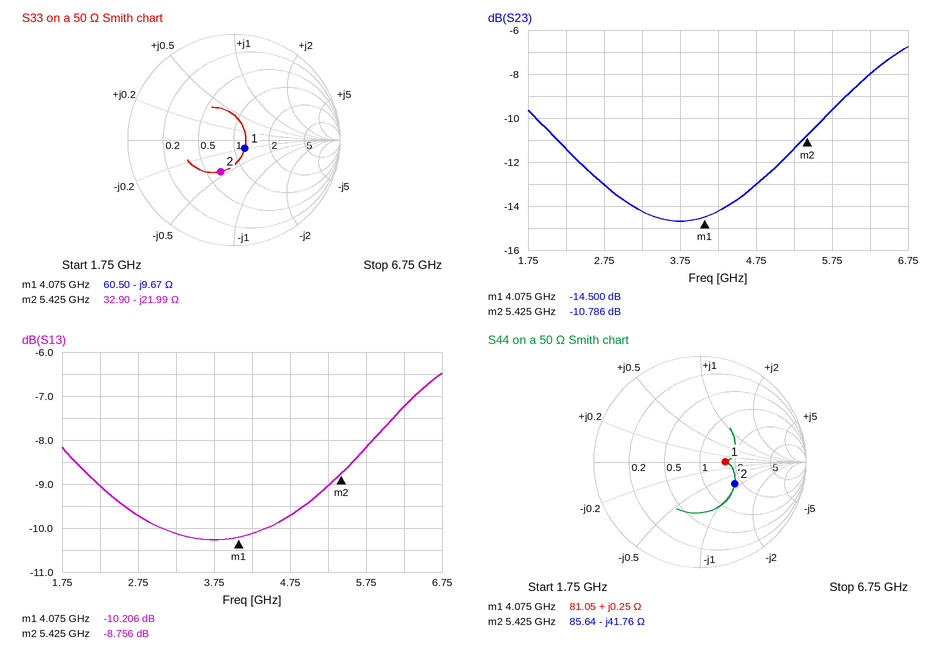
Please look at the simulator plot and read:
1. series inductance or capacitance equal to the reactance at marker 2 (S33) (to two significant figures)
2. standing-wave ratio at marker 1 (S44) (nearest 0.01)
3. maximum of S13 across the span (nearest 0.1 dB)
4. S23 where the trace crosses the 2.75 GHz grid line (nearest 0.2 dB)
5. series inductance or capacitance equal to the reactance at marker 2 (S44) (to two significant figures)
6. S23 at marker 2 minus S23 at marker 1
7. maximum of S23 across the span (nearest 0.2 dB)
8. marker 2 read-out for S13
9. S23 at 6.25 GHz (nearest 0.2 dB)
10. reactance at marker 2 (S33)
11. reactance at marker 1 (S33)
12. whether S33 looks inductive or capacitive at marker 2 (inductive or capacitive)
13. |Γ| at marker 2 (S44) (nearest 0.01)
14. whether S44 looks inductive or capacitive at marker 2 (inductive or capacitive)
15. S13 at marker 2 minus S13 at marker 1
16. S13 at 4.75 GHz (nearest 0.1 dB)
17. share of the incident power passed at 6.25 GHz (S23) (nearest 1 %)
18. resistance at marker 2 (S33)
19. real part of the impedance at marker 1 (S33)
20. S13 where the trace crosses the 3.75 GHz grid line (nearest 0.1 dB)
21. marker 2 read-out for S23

1.3 pF
1.62
-6.5 dB
-13.0 dB
700 fF
3.714 dB
-6.8 dB
-8.756 dB
-8.0 dB
-21.99 Ω
-9.67 Ω
capacitive
0.39
capacitive
1.450 dB
-9.7 dB
16 %
32.90 Ω
60.50 Ω
-10.3 dB
-10.786 dB
